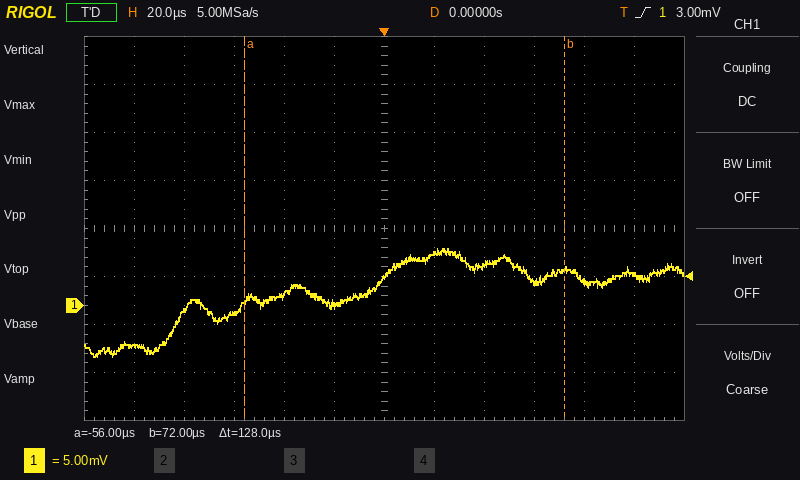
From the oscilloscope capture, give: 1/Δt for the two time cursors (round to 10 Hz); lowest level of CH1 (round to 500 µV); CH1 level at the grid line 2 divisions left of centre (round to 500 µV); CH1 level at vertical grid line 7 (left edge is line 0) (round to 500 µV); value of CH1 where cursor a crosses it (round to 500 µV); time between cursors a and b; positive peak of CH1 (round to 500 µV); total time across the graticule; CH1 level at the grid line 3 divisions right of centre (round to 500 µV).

7.81 kHz
-5.5 mV
1.0 mV
5.5 mV
500 µV
128 µs
6.0 mV
240 µs
2.5 mV
